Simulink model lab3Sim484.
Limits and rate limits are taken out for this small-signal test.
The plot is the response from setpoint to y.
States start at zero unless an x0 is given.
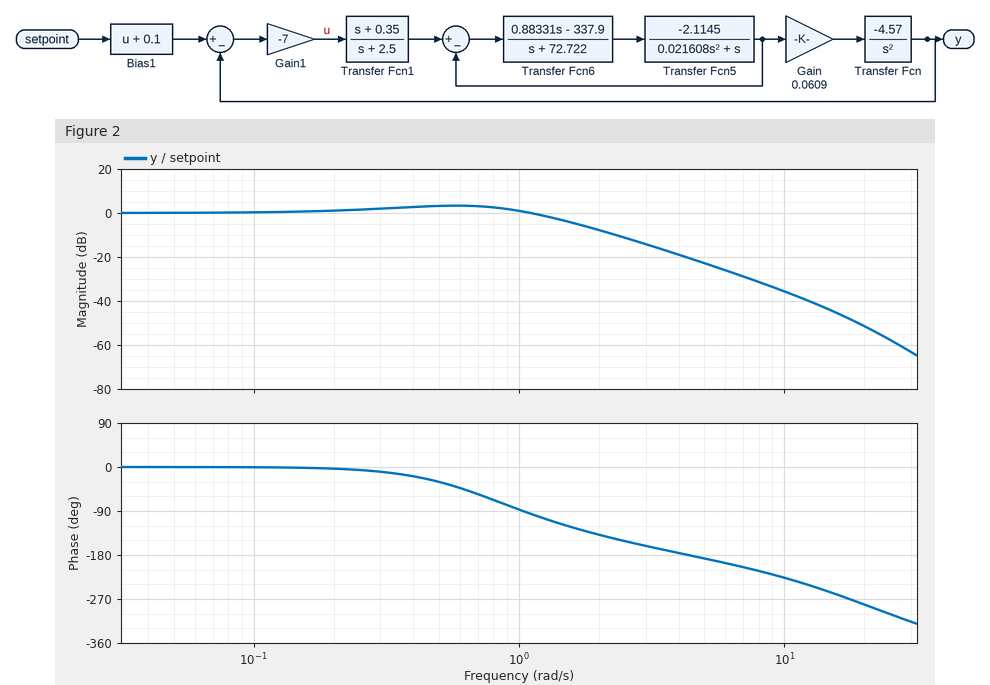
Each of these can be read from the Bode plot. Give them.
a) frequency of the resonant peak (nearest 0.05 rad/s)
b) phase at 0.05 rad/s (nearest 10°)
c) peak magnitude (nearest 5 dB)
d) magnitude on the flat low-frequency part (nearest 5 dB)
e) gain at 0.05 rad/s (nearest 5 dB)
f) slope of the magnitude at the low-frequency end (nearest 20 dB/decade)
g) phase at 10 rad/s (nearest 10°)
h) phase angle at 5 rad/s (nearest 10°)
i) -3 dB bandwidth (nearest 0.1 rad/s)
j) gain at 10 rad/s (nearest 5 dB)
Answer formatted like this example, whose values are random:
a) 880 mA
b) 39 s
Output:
a) 0.55 rad/s
b) 0°
c) 5 dB
d) 0 dB
e) 0 dB
f) 0 dB/decade
g) -230°
h) -190°
i) 1.4 rad/s
j) -35 dB
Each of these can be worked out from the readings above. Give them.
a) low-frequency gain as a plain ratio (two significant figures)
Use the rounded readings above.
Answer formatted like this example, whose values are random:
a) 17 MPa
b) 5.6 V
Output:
a) 1.0
